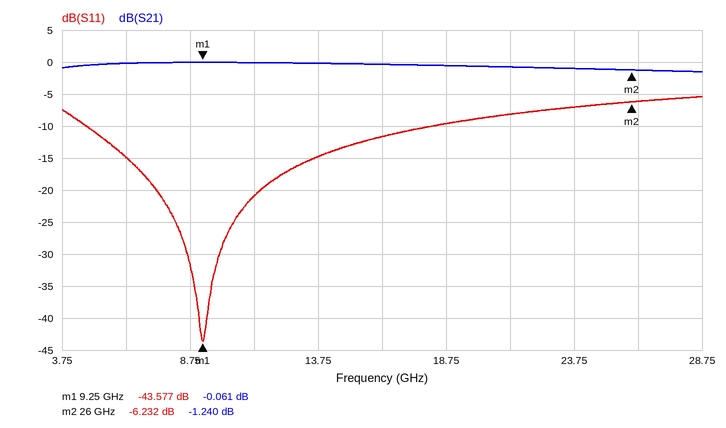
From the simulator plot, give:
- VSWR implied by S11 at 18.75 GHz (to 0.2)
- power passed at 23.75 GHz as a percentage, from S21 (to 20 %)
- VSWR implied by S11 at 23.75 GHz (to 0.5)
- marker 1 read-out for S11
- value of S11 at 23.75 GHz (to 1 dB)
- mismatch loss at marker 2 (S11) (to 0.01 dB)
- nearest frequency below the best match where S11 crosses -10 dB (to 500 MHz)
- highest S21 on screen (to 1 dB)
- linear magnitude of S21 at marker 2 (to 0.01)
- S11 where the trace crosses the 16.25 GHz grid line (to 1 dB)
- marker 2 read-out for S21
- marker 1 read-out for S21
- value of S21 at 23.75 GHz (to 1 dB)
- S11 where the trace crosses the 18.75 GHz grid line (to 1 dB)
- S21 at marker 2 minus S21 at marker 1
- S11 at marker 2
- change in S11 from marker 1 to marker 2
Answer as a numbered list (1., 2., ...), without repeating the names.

1. 2.0
2. 80 %
3. 2.5
4. -43.577 dB
5. -7 dB
6. 1.18 dB
7. 4.5 GHz
8. 0 dB
9. 0.87
10. -12 dB
11. -1.240 dB
12. -0.061 dB
13. -1 dB
14. -10 dB
15. -1.179 dB
16. -6.232 dB
17. 37.345 dB
